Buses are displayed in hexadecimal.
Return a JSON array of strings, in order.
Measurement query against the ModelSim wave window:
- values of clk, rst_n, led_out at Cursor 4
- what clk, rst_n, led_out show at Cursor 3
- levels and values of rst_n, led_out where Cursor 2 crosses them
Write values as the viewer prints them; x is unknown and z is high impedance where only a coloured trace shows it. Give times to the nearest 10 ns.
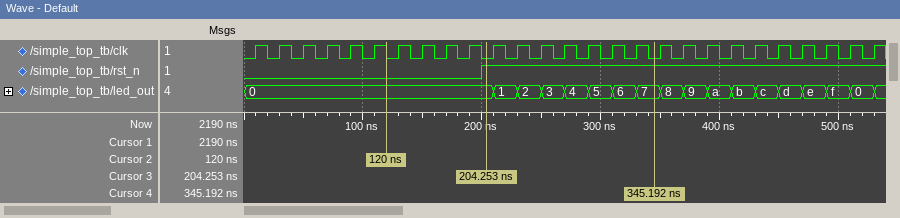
["clk=0, rst_n=1, led_out=7", "clk=0, rst_n=1, led_out=0", "rst_n=0, led_out=0"]
